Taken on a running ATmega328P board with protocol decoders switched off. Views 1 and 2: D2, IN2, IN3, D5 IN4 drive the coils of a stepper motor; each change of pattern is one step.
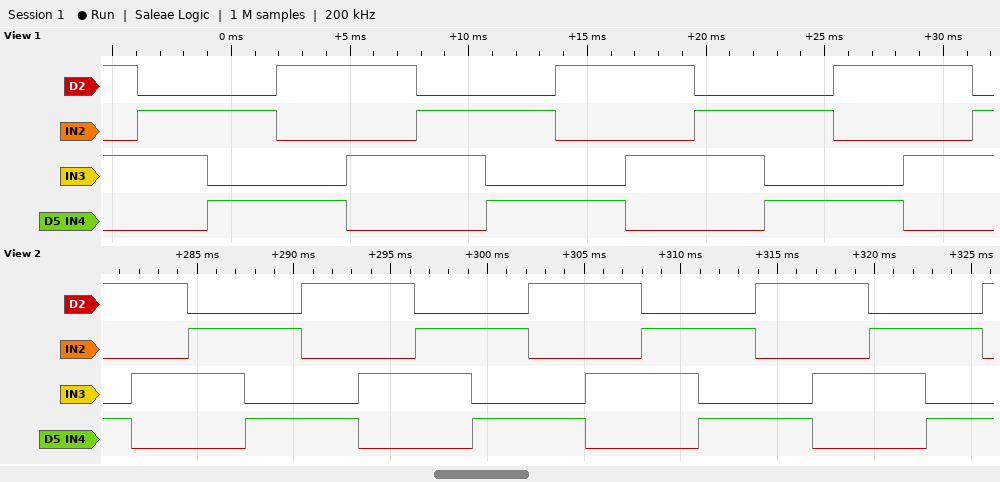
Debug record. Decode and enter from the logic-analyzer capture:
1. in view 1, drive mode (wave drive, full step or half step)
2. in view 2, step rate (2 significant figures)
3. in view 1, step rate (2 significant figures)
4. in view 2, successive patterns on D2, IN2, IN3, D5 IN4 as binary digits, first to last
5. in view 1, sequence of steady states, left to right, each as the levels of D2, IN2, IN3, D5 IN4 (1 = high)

full step
340 steps/s
340 steps/s
1001 1010 0110 0101 1001 1010 0110 0101 1001 1010 0110 0101 1001 1010 0110 0101 1001
1010 0110 0101 1001 1010 0110 0101 1001 1010 0110 0101 1001 1010 0110
